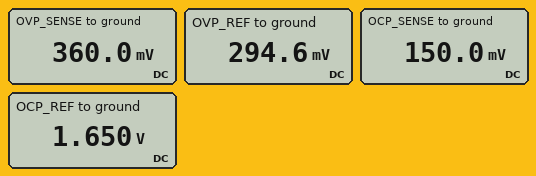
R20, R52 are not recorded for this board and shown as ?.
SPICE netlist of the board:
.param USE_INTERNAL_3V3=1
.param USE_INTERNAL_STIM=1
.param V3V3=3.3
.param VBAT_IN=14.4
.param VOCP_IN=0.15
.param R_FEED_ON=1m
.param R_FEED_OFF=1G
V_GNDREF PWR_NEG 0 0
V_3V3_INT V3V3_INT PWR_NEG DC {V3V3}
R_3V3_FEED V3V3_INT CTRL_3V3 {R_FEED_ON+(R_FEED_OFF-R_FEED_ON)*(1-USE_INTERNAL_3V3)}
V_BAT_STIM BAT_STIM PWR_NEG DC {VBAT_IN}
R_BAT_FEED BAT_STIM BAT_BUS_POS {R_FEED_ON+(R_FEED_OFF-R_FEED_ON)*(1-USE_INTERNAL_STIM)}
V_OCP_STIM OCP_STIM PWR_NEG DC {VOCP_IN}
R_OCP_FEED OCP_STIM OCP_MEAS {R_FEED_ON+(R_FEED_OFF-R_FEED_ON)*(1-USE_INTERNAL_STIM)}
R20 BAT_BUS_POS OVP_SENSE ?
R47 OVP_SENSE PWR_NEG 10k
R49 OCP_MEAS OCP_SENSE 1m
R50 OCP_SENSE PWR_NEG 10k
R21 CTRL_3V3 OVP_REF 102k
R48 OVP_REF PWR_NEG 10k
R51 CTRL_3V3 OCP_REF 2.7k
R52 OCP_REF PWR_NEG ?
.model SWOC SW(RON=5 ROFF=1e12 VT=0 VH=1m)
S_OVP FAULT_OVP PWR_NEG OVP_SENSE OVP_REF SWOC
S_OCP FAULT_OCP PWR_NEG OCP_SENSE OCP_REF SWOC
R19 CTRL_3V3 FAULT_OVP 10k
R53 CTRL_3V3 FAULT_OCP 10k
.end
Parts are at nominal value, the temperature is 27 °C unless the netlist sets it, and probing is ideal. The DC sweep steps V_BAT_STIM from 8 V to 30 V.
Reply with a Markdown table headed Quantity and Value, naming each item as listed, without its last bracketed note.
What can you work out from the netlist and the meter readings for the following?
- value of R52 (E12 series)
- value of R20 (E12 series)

| Quantity | Value |
|---|---|
| value of R52 | 2.7 kΩ |
| value of R20 | 390 kΩ |
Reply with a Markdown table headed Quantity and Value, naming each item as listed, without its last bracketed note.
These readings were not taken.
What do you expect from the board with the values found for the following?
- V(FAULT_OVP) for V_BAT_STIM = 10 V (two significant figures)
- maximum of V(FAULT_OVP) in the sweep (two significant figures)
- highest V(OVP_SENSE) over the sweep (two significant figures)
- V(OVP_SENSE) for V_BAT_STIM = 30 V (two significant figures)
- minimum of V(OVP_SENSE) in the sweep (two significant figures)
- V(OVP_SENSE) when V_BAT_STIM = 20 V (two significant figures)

| Quantity | Value |
|---|---|
| V(FAULT_OVP) for V_BAT_STIM = 10 V | 3.3 V |
| maximum of V(FAULT_OVP) in the sweep | 3.3 V |
| highest V(OVP_SENSE) over the sweep | 750 mV |
| V(OVP_SENSE) for V_BAT_STIM = 30 V | 750 mV |
| minimum of V(OVP_SENSE) in the sweep | 200 mV |
| V(OVP_SENSE) when V_BAT_STIM = 20 V | 500 mV |
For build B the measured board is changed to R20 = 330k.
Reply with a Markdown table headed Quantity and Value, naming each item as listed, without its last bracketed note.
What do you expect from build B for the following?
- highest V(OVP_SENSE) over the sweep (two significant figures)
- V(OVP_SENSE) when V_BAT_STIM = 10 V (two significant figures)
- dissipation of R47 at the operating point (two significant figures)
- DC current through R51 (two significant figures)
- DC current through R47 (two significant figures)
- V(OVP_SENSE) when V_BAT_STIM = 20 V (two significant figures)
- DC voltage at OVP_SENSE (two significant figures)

| Quantity | Value |
|---|---|
| highest V(OVP_SENSE) over the sweep | 880 mV |
| V(OVP_SENSE) when V_BAT_STIM = 10 V | 290 mV |
| dissipation of R47 at the operating point | 18 µW |
| DC current through R51 | 610 µA |
| DC current through R47 | 42 µA |
| V(OVP_SENSE) when V_BAT_STIM = 20 V | 590 mV |
| DC voltage at OVP_SENSE | 420 mV |
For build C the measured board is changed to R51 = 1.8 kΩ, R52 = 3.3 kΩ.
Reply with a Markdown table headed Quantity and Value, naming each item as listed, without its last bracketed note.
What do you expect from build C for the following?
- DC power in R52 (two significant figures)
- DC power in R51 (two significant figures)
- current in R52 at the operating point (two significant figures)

| Quantity | Value |
|---|---|
| DC power in R52 | 1.4 mW |
| DC power in R51 | 750 µW |
| current in R52 at the operating point | 650 µA |
